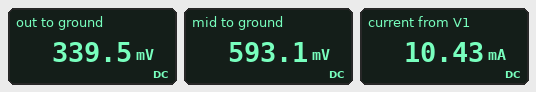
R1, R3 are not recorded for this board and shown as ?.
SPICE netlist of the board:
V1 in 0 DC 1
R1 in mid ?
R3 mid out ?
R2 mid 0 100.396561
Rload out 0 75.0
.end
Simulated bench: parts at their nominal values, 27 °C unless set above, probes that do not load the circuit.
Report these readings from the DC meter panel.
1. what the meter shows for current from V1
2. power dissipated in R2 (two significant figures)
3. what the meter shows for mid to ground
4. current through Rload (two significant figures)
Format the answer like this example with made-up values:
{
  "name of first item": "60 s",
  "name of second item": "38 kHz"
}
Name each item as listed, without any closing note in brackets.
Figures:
{
  "what the meter shows for current from V1": "10.43 mA",
  "power dissipated in R2": "3.5 mW",
  "what the meter shows for mid to ground": "593.1 mV",
  "current through Rload": "4.5 mA"
}
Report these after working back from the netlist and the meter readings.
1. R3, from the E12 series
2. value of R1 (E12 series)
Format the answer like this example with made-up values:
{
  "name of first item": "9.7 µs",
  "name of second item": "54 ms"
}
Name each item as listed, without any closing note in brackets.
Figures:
{
  "R3, from the E12 series": "56 Ω",
  "value of R1": "39 Ω"
}
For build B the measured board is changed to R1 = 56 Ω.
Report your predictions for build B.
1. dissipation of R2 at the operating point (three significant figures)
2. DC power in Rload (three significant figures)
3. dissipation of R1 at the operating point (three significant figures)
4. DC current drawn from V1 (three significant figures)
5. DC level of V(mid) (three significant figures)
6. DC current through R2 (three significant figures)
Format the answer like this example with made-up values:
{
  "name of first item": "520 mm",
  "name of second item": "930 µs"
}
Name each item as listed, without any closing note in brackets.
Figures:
{
  "dissipation of R2 at the operating point": "2.53 mW",
  "DC power in Rload": "1.11 mW",
  "dissipation of R1 at the operating point": "4.40 mW",
  "DC current drawn from V1": "8.86 mA",
  "DC level of V(mid)": "504 mV",
  "DC current through R2": "5.02 mA"
}
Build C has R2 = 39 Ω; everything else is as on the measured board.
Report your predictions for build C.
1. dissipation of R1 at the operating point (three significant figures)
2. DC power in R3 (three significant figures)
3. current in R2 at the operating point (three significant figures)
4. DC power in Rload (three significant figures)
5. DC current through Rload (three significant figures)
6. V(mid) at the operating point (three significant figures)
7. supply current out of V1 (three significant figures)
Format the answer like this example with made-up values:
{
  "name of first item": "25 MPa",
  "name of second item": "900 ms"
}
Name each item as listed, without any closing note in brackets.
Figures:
{
  "dissipation of R1 at the operating point": "8.18 mW",
  "DC power in R3": "618 µW",
  "current in R2 at the operating point": "11.2 mA",
  "DC power in Rload": "828 µW",
  "DC current through Rload": "3.32 mA",
  "V(mid) at the operating point": "435 mV",
  "supply current out of V1": "14.5 mA"
}
